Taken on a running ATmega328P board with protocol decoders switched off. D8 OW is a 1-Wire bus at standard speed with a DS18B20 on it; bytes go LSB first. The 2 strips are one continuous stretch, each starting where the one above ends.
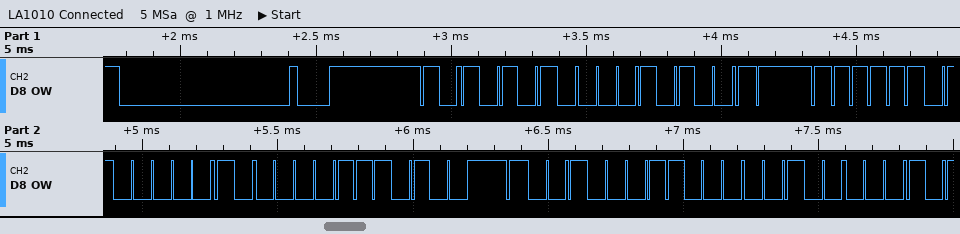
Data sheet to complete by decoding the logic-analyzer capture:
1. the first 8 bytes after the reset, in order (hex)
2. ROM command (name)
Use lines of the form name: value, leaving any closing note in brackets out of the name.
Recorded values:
the first 8 bytes after the reset, in order: 55 28 FF 82 E0 92 18 04
ROM command: Match ROM
